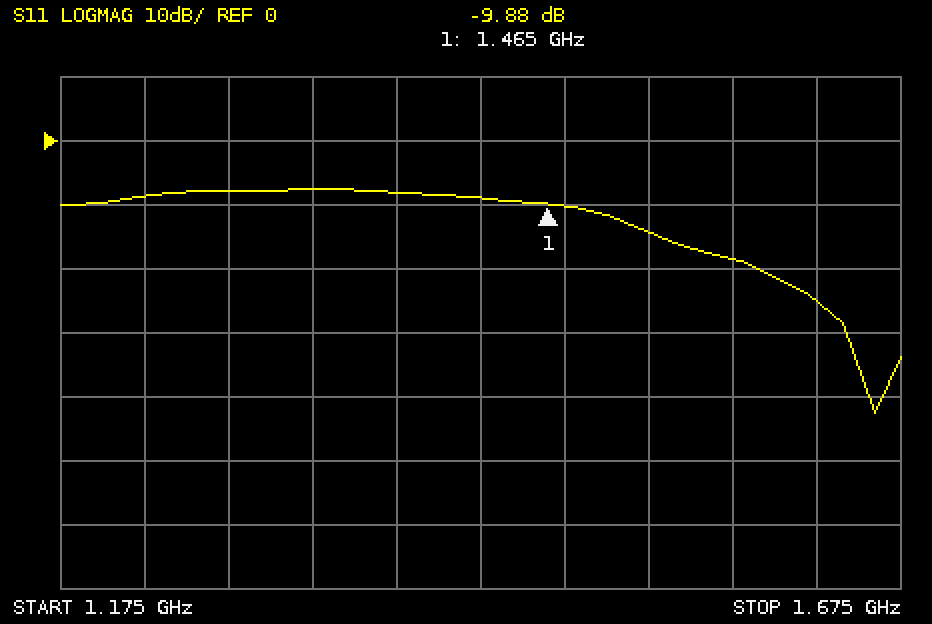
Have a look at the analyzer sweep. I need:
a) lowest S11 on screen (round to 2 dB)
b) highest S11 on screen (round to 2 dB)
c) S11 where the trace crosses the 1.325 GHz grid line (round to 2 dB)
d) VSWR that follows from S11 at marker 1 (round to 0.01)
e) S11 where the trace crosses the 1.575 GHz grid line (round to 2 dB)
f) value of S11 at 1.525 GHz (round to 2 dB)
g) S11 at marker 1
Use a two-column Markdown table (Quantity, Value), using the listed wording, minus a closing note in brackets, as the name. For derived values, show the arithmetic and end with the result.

| Quantity | Value |
|---|---|
| lowest S11 on screen | -42 dB |
| highest S11 on screen | -8 dB |
| S11 where the trace crosses the 1.325 GHz grid line | -8 dB |
| VSWR that follows from S11 at marker 1 | (1 + 0.3206)/(1 − 0.3206) ≈ 1.94 |
| S11 where the trace crosses the 1.575 GHz grid line | -18 dB |
| value of S11 at 1.525 GHz | -14 dB |
| S11 at marker 1 | -9.88 dB |
